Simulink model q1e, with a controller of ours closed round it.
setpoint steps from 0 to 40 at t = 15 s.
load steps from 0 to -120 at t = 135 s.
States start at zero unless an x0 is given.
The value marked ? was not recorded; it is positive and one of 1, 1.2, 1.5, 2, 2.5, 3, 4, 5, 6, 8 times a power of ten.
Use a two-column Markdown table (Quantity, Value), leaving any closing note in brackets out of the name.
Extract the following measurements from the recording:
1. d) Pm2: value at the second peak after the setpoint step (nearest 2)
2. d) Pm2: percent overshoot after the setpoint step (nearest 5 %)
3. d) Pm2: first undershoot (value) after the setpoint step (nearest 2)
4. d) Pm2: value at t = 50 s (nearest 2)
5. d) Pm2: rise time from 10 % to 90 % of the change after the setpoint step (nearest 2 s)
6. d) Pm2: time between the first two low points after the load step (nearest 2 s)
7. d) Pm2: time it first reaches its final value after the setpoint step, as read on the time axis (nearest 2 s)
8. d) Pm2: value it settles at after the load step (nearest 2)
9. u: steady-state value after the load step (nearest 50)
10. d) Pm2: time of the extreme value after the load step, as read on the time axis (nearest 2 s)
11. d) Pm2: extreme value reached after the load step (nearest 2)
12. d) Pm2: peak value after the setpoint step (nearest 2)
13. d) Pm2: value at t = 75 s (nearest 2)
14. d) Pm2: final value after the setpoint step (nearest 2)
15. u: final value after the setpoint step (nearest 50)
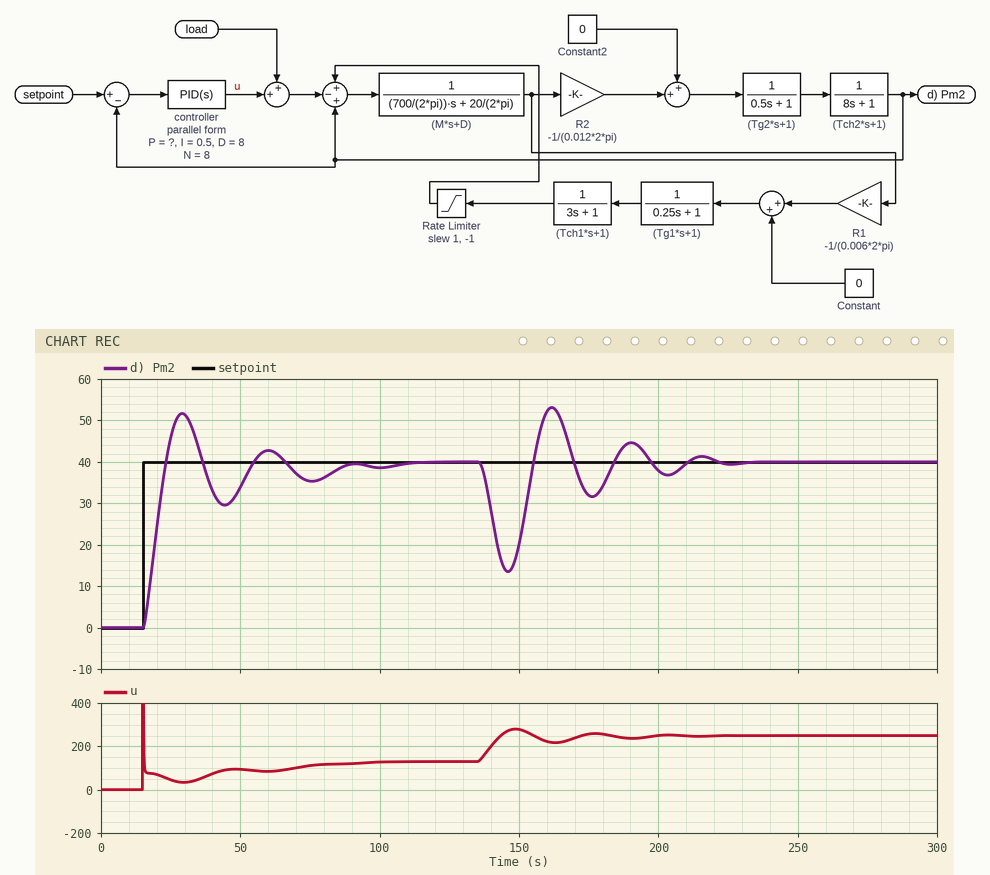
| Quantity | Value |
|---|---|
| d) Pm2: value at the second peak after the setpoint step | 42 |
| d) Pm2: percent overshoot after the setpoint step | 30 % |
| d) Pm2: first undershoot (value) after the setpoint step | 30 |
| d) Pm2: value at t = 50 s | 34 |
| d) Pm2: rise time from 10 % to 90 % of the change after the setpoint step | 6 s |
| d) Pm2: time between the first two low points after the load step | 30 s |
| d) Pm2: time it first reaches its final value after the setpoint step, as read on the time axis | 24 s |
| d) Pm2: value it settles at after the load step | 40 |
| u: steady-state value after the load step | 250 |
| d) Pm2: time of the extreme value after the load step, as read on the time axis | 146 s |
| d) Pm2: extreme value reached after the load step | 14 |
| d) Pm2: peak value after the setpoint step | 52 |
| d) Pm2: value at t = 75 s | 36 |
| d) Pm2: final value after the setpoint step | 40 |
| u: final value after the setpoint step | 150 |
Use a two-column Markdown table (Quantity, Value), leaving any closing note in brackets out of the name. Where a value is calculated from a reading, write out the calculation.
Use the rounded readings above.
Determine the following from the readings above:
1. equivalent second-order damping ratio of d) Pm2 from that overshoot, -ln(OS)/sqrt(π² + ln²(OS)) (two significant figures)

| Quantity | Value |
|---|---|
| equivalent second-order damping ratio of d) Pm2 from that overshoot, -ln(OS)/sqrt(π² + ln²(OS)) | ln(0.3) = -1.204; 1.204 / sqrt(9.870 + 1.450) = 0.36 |
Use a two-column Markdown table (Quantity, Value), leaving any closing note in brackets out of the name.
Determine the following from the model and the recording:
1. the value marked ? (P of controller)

| Quantity | Value |
|---|---|
| the value marked ? | 2.5 |
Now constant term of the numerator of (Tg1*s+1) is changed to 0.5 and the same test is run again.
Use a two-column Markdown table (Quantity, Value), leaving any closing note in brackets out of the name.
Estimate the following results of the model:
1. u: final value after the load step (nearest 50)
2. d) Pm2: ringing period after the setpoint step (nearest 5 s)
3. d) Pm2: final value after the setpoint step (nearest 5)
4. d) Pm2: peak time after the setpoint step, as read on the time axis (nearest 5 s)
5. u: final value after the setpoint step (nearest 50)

| Quantity | Value |
|---|---|
| u: final value after the load step | 200 |
| d) Pm2: ringing period after the setpoint step | 30 s |
| d) Pm2: final value after the setpoint step | 40 |
| d) Pm2: peak time after the setpoint step, as read on the time axis | 30 s |
| u: final value after the setpoint step | 100 |
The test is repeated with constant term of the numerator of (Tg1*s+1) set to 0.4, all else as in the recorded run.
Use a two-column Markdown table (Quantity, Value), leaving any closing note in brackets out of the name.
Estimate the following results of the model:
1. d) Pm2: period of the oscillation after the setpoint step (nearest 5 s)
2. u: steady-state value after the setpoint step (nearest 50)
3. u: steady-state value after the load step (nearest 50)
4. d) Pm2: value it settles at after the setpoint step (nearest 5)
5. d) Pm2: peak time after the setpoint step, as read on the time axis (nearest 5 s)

| Quantity | Value |
|---|---|
| d) Pm2: period of the oscillation after the setpoint step | 30 s |
| u: steady-state value after the setpoint step | 100 |
| u: steady-state value after the load step | 200 |
| d) Pm2: value it settles at after the setpoint step | 40 |
| d) Pm2: peak time after the setpoint step, as read on the time axis | 30 s |
